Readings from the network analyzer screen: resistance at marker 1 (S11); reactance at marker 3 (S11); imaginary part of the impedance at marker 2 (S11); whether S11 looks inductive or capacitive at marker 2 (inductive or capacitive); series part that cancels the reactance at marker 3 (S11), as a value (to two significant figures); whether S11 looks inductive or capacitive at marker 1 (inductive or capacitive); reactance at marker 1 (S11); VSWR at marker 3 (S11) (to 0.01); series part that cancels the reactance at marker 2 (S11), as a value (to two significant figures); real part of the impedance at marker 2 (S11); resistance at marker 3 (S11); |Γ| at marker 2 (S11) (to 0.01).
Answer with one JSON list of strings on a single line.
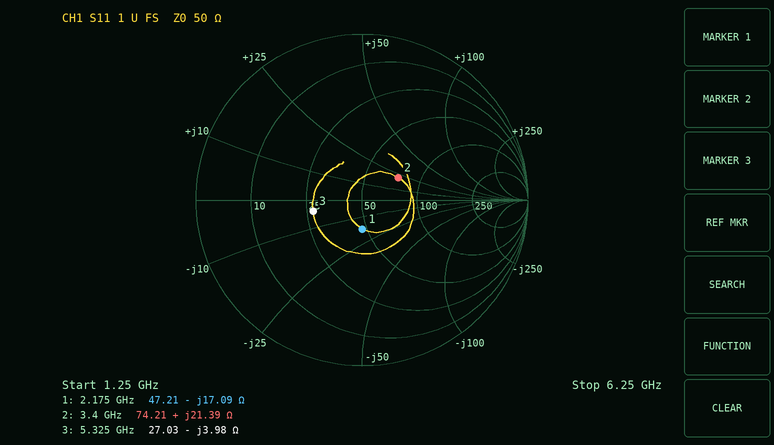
["47.21 Ω", "-3.98 Ω", "+21.39 Ω", "inductive", "120 pH", "capacitive", "-17.09 Ω", "1.87", "2.2 pF", "74.21 Ω", "27.03 Ω", "0.26"]
